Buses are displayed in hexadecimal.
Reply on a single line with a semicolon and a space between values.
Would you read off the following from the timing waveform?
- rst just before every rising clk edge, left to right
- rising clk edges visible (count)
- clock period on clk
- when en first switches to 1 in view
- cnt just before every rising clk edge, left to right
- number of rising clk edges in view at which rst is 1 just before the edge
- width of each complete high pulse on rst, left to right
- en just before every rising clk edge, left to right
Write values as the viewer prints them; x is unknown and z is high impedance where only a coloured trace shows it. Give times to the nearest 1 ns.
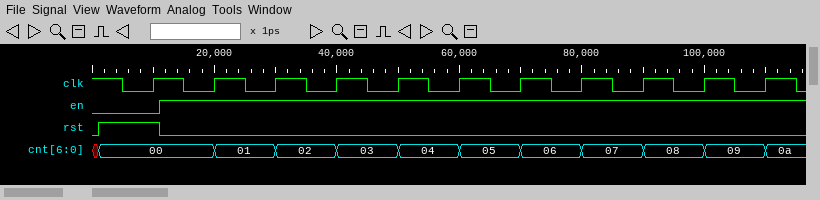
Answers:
1 0 0 0 0 0 0 0 0 0 0; 11; 10 ns; 11 ns; 00, 00, 01, 02, 03, 04, 05, 06, 07, 08, 09; 1; 10 ns; 0 1 1 1 1 1 1 1 1 1 1
